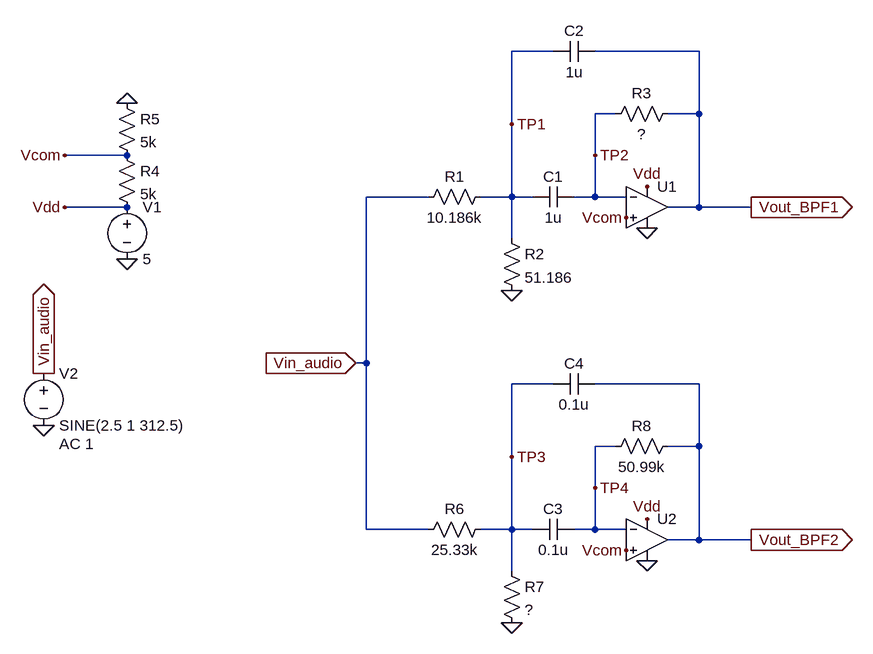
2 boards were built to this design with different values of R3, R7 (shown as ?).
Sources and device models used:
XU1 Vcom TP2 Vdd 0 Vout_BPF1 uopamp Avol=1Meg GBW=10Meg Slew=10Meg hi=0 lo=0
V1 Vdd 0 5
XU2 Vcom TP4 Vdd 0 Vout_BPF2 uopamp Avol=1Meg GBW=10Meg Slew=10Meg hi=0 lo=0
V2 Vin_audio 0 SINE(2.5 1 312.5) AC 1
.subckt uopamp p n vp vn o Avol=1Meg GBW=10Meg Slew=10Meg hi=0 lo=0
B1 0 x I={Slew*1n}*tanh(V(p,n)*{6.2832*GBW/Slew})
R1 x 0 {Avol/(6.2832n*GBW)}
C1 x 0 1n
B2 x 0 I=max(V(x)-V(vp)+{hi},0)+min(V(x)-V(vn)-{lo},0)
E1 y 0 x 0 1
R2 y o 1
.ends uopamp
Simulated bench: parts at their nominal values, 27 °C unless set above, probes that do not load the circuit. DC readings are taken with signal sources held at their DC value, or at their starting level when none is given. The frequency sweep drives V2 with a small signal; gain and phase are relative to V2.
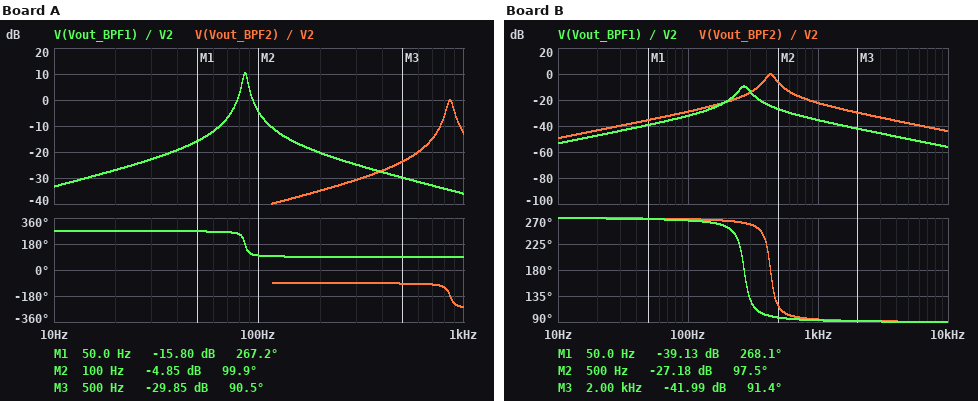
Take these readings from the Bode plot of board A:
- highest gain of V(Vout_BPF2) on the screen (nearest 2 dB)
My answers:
0 dB
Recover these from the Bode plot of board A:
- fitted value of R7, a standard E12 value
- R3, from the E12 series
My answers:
68 Ω
68 kΩ
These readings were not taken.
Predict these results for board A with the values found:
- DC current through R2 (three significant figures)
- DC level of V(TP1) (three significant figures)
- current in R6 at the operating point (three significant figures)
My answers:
244 µA
12.5 mV
98.4 µA
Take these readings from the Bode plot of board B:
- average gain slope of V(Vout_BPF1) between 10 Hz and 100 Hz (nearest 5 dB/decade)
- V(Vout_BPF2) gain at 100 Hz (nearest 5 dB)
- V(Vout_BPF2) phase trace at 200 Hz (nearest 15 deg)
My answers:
20 dB/decade
-30 dB
270 deg
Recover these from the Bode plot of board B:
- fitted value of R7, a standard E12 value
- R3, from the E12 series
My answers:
270 Ω
6.8 kΩ
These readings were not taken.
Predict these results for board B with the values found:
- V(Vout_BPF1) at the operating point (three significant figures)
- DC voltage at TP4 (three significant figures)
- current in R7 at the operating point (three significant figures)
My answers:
2.50 V
2.50 V
97.7 µA
